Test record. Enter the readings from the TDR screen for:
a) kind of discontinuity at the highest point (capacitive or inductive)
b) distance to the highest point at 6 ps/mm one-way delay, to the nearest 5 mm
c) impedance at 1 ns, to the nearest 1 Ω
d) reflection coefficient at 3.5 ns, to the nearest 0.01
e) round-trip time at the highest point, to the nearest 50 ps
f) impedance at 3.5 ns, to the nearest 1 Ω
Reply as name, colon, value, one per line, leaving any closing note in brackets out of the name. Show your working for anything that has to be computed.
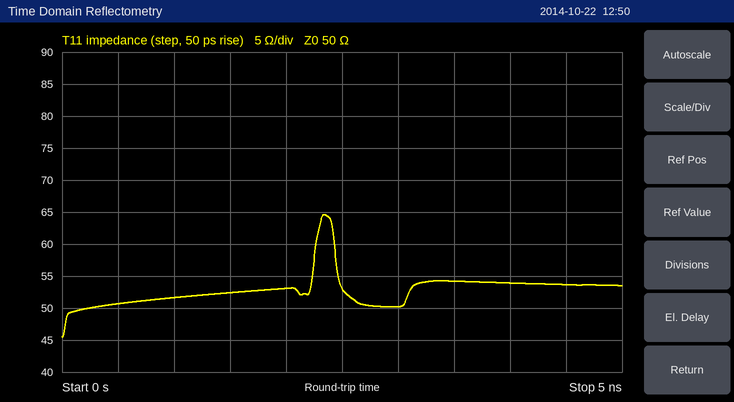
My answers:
kind of discontinuity at the highest point: inductive
distance to the highest point at 6 ps/mm one-way delay, to the nearest 5 mm: 2.35 ns / 2 / 6 ps/mm ≈ 196 mm, so 195 mm to the nearest 5 mm
impedance at 1 ns, to the nearest 1 Ω: 52 Ω
reflection coefficient at 3.5 ns, to the nearest 0.01: (54 − 50)/(54 + 50) ≈ +0.04
round-trip time at the highest point, to the nearest 50 ps: 2.35 ns
impedance at 3.5 ns, to the nearest 1 Ω: 54 Ω
